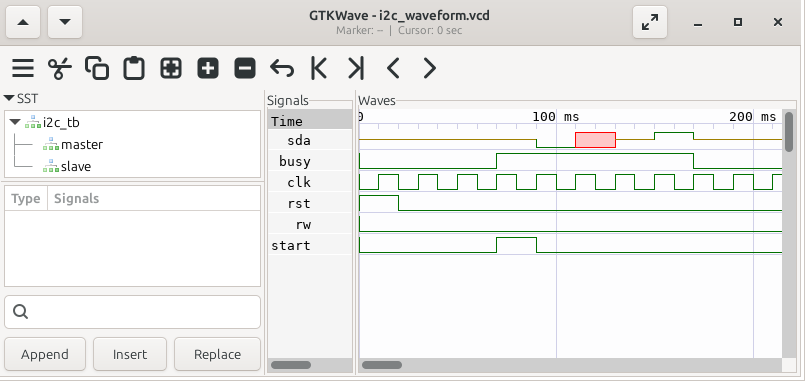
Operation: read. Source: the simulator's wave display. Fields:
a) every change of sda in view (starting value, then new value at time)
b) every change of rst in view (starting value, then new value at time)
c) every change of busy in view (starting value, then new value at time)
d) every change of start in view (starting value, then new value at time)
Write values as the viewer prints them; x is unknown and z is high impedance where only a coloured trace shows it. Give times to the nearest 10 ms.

z, 0 at 90 ms, x at 110 ms, z at 130 ms, 1 at 150 ms, z at 170 ms
1, 0 at 20 ms
0, 1 at 70 ms, 0 at 170 ms
0, 1 at 70 ms, 0 at 90 ms
